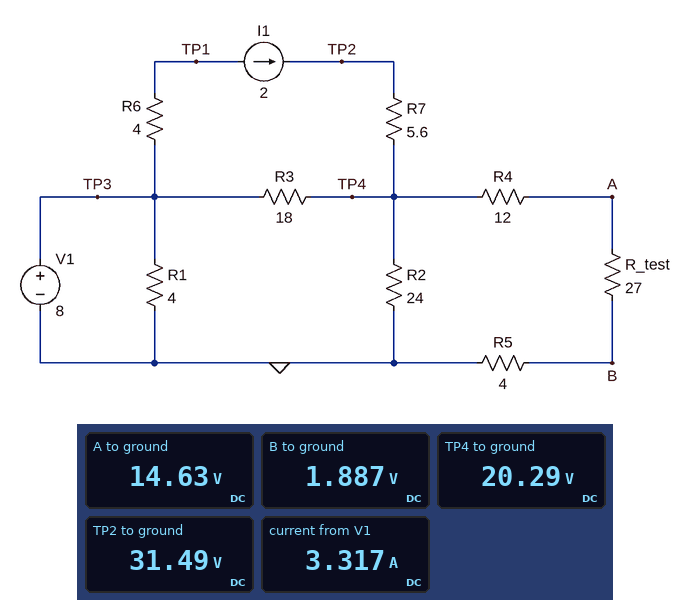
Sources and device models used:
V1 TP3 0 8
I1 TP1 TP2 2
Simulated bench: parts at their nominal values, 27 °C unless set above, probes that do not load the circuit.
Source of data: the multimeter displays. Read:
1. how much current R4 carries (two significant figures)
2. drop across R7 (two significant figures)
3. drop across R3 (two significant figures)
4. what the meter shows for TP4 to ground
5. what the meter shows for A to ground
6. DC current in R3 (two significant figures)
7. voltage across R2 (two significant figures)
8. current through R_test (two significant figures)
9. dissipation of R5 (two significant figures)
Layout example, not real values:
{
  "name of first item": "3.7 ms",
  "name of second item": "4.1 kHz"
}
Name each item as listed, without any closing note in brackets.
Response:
{
  "how much current R4 carries": "470 mA",
  "drop across R7": "11 V",
  "drop across R3": "12 V",
  "what the meter shows for TP4 to ground": "20.29 V",
  "what the meter shows for A to ground": "14.63 V",
  "DC current in R3": "680 mA",
  "voltage across R2": "20 V",
  "current through R_test": "470 mA",
  "dissipation of R5": "890 mW"
}
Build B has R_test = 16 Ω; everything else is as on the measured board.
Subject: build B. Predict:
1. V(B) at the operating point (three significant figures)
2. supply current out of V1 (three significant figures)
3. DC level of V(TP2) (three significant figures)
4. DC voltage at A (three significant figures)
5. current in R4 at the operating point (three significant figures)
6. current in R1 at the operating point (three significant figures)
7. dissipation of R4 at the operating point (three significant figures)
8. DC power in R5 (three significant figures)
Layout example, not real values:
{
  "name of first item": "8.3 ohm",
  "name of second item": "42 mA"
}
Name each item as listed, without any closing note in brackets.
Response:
{
  "V(B) at the operating point": "2.38 V",
  "supply current out of V1": "3.39 A",
  "DC level of V(TP2)": "30.2 V",
  "DC voltage at A": "11.9 V",
  "current in R4 at the operating point": "595 mA",
  "current in R1 at the operating point": "2.00 A",
  "dissipation of R4 at the operating point": "4.24 W",
  "DC power in R5": "1.41 W"
}
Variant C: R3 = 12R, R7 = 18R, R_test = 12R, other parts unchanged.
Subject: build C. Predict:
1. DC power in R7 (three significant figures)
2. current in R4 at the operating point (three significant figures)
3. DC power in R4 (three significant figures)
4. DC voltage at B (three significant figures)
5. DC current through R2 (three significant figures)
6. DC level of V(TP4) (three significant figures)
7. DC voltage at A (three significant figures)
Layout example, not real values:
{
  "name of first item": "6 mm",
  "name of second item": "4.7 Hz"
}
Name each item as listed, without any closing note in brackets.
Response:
{
  "DC power in R7": "72.0 W",
  "current in R4 at the operating point": "593 mA",
  "DC power in R4": "4.21 W",
  "DC voltage at B": "2.37 V",
  "DC current through R2": "691 mA",
  "DC level of V(TP4)": "16.6 V",
  "DC voltage at A": "9.48 V"
}
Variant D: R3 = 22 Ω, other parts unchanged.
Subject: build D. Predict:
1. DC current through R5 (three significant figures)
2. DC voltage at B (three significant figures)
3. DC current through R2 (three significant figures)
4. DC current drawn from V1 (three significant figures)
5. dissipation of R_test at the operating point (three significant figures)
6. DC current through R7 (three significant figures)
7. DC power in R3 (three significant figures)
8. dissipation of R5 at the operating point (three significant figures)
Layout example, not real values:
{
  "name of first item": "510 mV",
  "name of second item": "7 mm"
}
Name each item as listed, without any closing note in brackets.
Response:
{
  "DC current through R5": "498 mA",
  "DC voltage at B": "1.99 V",
  "DC current through R2": "892 mA",
  "DC current drawn from V1": "3.39 A",
  "dissipation of R_test at the operating point": "6.70 W",
  "DC current through R7": "2.00 A",
  "DC power in R3": "8.18 W",
  "dissipation of R5 at the operating point": "992 mW"
}
